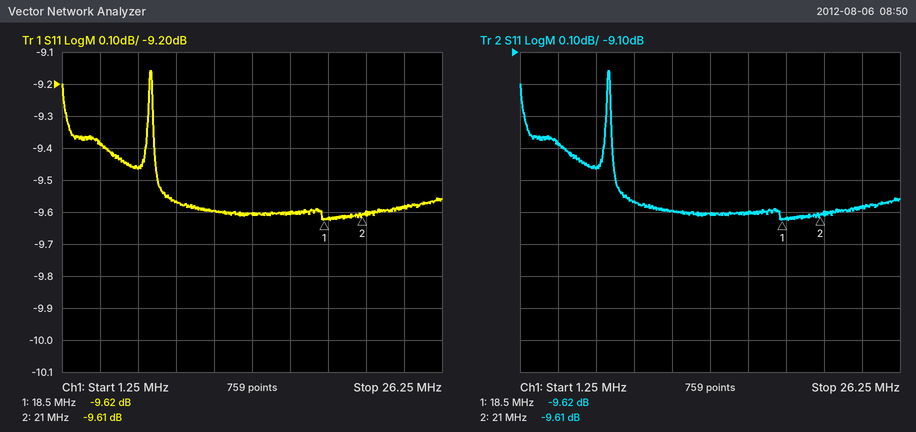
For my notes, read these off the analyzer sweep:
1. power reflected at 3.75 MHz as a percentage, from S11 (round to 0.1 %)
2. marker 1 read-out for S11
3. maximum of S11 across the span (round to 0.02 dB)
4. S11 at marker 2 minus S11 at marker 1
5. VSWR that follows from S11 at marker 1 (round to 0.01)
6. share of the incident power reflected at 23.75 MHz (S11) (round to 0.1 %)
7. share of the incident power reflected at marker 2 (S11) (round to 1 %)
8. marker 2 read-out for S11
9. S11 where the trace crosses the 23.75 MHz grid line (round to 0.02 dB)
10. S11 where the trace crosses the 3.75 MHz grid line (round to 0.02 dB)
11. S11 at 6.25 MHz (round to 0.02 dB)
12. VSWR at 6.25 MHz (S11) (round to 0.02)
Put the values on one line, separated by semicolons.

11.5 %; -9.62 dB; -9.16 dB; 0.01 dB; 1.99; 11.0 %; 11 %; -9.61 dB; -9.58 dB; -9.38 dB; -9.46 dB; 2.02
